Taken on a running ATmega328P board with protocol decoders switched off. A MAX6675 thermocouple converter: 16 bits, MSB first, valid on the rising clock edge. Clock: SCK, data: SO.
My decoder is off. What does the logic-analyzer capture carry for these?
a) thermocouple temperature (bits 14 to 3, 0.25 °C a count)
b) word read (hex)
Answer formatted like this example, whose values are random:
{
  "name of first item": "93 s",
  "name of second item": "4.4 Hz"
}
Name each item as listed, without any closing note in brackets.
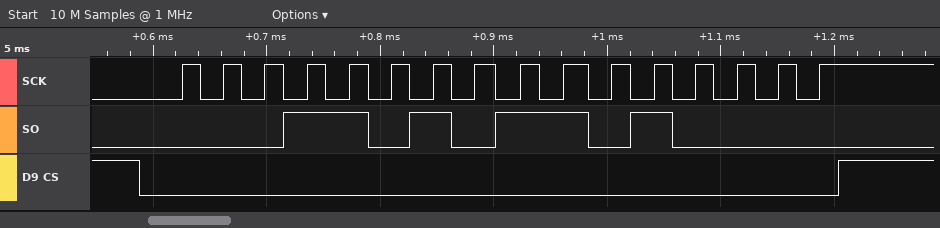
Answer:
{
  "thermocouple temperature": "214.50 °C",
  "word read": "0x1AD0"
}
